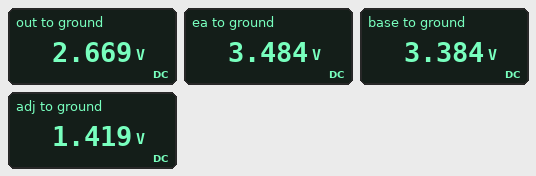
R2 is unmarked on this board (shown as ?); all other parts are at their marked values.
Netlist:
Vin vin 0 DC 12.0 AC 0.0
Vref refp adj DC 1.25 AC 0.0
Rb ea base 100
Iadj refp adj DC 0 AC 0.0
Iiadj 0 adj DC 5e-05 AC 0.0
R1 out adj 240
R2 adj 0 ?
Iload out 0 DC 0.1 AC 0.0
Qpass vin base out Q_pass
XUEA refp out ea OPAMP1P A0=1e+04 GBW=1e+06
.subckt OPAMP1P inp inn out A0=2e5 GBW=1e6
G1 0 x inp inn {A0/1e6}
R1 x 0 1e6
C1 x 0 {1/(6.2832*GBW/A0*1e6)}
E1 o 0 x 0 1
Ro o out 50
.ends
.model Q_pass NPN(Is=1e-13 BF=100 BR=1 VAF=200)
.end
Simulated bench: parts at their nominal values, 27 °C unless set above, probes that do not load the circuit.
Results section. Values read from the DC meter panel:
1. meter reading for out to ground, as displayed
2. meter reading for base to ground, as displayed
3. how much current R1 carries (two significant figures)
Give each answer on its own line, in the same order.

2.669 V
3.384 V
5.2 mA
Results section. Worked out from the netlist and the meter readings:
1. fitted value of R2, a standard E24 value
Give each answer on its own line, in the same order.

270 Ω
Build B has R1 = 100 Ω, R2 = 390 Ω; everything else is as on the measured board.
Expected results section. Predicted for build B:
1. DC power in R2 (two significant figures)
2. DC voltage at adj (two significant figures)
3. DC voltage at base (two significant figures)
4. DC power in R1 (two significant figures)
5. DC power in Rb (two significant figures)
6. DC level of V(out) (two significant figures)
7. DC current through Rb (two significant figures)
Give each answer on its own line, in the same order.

61 mW
4.9 V
6.9 V
16 mW
120 µW
6.1 V
1.1 mA
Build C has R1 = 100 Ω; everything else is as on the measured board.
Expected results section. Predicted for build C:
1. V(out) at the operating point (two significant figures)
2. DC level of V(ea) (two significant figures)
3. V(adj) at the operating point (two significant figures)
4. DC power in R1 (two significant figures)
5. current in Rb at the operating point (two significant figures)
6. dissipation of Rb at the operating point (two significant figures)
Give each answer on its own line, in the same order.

4.6 V
5.5 V
3.4 V
16 mW
1.1 mA
120 µW
